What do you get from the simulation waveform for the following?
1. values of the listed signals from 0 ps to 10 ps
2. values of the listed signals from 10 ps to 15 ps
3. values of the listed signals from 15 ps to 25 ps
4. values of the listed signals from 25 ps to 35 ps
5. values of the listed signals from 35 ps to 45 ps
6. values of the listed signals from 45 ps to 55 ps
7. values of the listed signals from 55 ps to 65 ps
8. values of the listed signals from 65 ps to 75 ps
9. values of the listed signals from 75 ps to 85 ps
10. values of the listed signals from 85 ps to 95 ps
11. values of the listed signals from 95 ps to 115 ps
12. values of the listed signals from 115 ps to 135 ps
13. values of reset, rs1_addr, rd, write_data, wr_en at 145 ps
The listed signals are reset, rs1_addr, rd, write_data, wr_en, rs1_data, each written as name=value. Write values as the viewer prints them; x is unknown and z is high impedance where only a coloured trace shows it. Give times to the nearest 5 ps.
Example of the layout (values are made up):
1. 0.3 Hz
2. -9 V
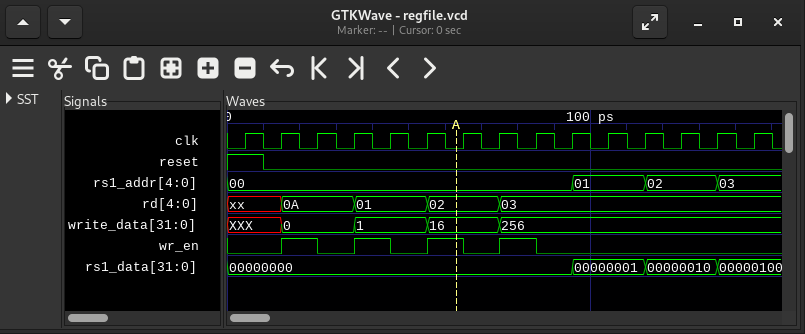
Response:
1. reset=1, rs1_addr=00, rd=xx, write_data=XXX, wr_en=0, rs1_data=00000000
2. reset=0, rs1_addr=00, rd=xx, write_data=XXX, wr_en=0, rs1_data=00000000
3. reset=0, rs1_addr=00, rd=0A, write_data=0, wr_en=1, rs1_data=00000000
4. reset=0, rs1_addr=00, rd=0A, write_data=0, wr_en=0, rs1_data=00000000
5. reset=0, rs1_addr=00, rd=01, write_data=1, wr_en=1, rs1_data=00000000
6. reset=0, rs1_addr=00, rd=01, write_data=1, wr_en=0, rs1_data=00000000
7. reset=0, rs1_addr=00, rd=02, write_data=16, wr_en=1, rs1_data=00000000
8. reset=0, rs1_addr=00, rd=02, write_data=16, wr_en=0, rs1_data=00000000
9. reset=0, rs1_addr=00, rd=03, write_data=256, wr_en=1, rs1_data=00000000
10. reset=0, rs1_addr=00, rd=03, write_data=256, wr_en=0, rs1_data=00000000
11. reset=0, rs1_addr=01, rd=03, write_data=256, wr_en=0, rs1_data=00000001
12. reset=0, rs1_addr=02, rd=03, write_data=256, wr_en=0, rs1_data=00000010
13. reset=0, rs1_addr=03, rd=03, write_data=256, wr_en=0
